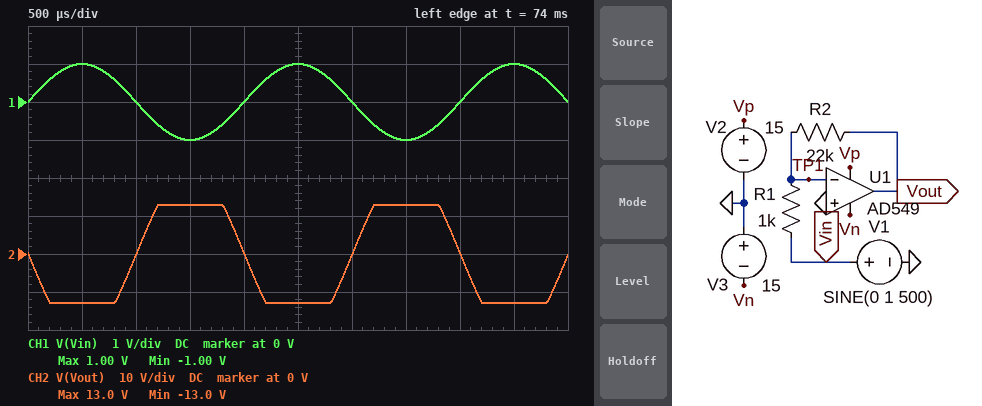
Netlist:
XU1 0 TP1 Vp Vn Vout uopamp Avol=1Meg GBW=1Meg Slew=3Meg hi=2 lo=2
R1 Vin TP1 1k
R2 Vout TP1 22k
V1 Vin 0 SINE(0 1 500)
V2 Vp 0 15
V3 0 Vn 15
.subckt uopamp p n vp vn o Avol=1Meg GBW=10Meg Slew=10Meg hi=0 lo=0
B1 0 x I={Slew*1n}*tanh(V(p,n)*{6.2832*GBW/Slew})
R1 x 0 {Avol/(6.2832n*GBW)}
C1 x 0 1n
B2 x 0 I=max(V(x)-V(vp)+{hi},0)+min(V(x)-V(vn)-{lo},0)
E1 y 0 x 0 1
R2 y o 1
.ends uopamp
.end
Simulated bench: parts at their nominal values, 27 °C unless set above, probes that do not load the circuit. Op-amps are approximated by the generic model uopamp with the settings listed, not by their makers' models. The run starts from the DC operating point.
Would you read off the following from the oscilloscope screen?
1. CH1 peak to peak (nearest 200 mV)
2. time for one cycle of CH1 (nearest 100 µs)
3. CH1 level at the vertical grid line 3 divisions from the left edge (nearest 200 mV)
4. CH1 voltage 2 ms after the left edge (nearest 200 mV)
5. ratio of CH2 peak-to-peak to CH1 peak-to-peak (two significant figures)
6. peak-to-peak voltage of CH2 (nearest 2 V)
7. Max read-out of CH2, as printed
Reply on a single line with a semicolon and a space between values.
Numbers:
2.0 V; 2.0 ms; -1.0 V; 0 V; 13; 26 V; 13.0 V
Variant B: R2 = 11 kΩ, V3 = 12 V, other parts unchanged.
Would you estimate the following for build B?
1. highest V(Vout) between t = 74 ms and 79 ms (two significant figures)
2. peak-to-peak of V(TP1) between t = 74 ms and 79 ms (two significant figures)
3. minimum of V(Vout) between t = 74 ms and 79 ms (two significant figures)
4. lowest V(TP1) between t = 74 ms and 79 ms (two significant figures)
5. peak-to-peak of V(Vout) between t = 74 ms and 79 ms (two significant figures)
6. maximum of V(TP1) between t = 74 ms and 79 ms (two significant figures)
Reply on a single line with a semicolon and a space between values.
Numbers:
11 V; 89 mV; -10 V; -5.5 mV; 21 V; 83 mV
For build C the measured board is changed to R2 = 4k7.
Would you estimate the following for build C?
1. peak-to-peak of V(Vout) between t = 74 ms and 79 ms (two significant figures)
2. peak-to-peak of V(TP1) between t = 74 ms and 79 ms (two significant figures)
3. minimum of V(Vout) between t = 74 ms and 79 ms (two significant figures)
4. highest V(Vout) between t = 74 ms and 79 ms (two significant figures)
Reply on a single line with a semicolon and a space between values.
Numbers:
9.4 V; 4.7 mV; -4.7 V; 4.7 V
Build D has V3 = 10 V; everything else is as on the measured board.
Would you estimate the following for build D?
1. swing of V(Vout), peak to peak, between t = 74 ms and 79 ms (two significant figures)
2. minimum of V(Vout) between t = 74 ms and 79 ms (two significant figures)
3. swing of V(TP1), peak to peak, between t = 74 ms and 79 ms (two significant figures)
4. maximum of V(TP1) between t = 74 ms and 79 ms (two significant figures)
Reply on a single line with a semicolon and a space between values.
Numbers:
21 V; -8.0 V; 1.0 V; 610 mV
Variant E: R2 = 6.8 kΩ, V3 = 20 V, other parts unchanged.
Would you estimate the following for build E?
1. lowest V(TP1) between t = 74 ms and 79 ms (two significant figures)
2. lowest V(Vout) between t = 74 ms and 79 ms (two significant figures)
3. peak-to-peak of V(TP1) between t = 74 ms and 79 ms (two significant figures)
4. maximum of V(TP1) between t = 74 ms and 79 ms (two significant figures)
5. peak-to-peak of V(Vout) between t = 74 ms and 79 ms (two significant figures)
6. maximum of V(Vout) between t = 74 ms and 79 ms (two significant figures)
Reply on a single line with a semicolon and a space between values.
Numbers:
-3.4 mV; -6.8 V; 6.8 mV; 3.4 mV; 14 V; 6.8 V
